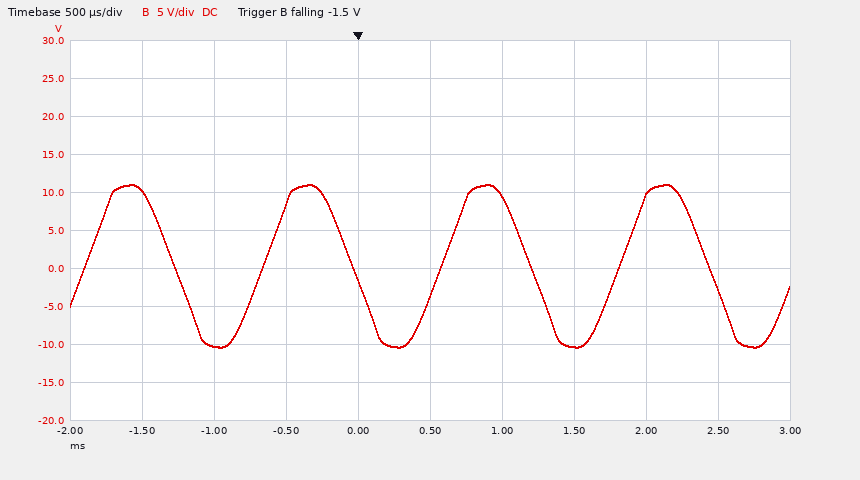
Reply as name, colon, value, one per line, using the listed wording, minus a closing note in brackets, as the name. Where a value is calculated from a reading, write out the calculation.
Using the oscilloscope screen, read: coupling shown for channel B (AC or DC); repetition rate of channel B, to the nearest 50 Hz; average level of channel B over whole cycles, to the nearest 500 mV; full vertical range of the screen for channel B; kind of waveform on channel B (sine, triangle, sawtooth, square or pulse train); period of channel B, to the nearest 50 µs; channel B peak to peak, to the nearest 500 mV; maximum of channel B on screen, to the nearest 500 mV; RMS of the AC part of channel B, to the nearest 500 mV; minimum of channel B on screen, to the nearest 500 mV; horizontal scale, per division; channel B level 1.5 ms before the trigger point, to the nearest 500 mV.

coupling shown for channel B: DC
repetition rate of channel B, to the nearest 50 Hz: 1 / 1.25 ms ≈ 800 Hz
average level of channel B over whole cycles, to the nearest 500 mV: (11.0 V + (-10.5 V)) / 2 ≈ 250 mV, so 500 mV to the nearest 500 mV
full vertical range of the screen for channel B: 50 V
kind of waveform on channel B: sine
period of channel B, to the nearest 50 µs: 1.25 ms
channel B peak to peak, to the nearest 500 mV: 11.0 V − (-10.5 V) = 21.5 V
maximum of channel B on screen, to the nearest 500 mV: 11.0 V
RMS of the AC part of channel B, to the nearest 500 mV: 21.5 V / (2√2) ≈ 7.60 V, so 7.5 V to the nearest 500 mV
minimum of channel B on screen, to the nearest 500 mV: -10.5 V
horizontal scale, per division: 500 µs
channel B level 1.5 ms before the trigger point, to the nearest 500 mV: 10.0 V
